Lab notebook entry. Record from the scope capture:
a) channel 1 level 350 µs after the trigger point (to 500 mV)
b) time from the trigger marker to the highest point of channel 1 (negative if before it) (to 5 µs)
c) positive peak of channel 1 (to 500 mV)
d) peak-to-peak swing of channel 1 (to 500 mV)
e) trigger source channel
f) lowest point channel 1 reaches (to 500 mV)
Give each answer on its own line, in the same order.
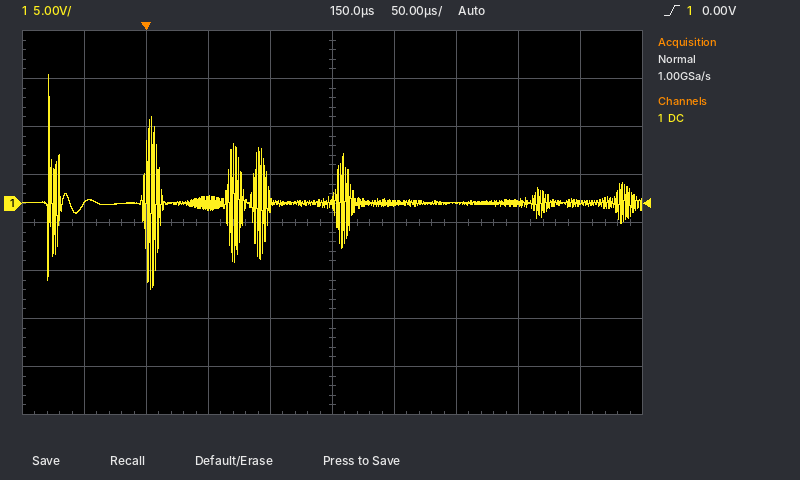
0.0 V
-80 µs
13.5 V
22.5 V
channel 1
-9.0 V
